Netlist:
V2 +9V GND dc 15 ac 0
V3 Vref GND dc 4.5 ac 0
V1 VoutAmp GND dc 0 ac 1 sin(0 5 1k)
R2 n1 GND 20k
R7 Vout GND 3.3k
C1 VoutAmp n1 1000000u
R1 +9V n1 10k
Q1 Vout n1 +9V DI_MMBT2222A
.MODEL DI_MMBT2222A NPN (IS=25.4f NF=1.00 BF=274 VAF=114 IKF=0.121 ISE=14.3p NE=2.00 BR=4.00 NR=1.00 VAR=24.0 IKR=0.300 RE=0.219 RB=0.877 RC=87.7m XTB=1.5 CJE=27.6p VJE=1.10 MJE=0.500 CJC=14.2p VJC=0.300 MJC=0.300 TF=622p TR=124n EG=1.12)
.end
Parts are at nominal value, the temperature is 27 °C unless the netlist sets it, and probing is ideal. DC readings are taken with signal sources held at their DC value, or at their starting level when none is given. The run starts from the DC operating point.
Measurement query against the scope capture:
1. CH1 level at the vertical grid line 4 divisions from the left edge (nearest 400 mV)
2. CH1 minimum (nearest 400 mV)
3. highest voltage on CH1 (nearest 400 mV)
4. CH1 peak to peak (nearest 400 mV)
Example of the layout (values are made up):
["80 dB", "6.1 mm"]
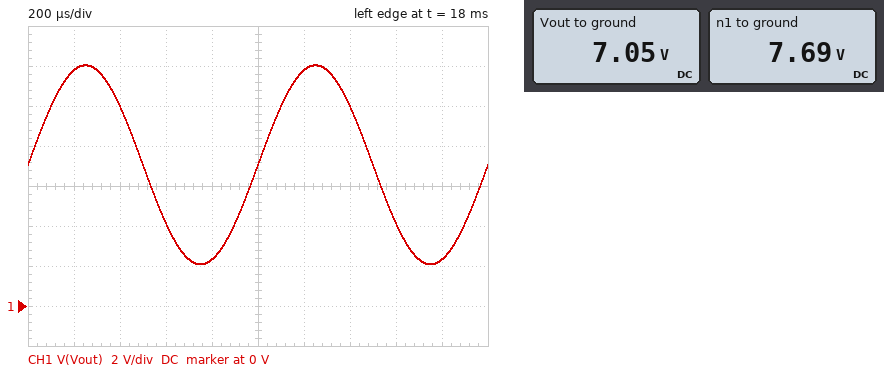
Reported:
["2.4 V", "2.0 V", "12.0 V", "10.0 V"]
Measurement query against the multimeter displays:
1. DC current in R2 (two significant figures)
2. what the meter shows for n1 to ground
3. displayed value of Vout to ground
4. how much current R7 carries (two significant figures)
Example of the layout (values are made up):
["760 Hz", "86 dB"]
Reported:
["380 µA", "7.69 V", "7.05 V", "2.1 mA"]
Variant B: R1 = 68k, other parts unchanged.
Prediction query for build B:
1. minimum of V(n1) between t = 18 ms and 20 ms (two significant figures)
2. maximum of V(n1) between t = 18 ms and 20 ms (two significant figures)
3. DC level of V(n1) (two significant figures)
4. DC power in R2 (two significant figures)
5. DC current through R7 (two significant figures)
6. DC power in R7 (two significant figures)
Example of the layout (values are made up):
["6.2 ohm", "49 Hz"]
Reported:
["-2.7 V", "7.3 V", "2.3 V", "260 µW", "510 µA", "870 µW"]
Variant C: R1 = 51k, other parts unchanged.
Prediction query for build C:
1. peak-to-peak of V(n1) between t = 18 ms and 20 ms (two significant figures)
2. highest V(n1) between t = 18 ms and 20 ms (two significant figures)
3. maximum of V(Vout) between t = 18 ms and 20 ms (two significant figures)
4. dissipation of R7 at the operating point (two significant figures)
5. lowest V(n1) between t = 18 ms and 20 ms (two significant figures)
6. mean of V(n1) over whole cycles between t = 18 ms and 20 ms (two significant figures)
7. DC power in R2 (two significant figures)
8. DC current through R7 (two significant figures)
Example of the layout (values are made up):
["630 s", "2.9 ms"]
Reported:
["10 V", "7.8 V", "7.2 V", "1.5 mW", "-2.2 V", "2.8 V", "400 µW", "680 µA"]
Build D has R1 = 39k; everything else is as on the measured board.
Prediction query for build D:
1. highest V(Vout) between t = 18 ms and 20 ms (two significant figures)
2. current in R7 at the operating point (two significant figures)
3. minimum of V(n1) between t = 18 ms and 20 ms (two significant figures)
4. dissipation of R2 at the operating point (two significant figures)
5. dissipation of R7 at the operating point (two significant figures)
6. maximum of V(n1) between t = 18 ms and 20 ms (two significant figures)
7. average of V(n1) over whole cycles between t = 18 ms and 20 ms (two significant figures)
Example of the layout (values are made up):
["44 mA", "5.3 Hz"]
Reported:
["7.8 V", "860 µA", "-1.6 V", "590 µW", "2.4 mW", "8.4 V", "3.4 V"]
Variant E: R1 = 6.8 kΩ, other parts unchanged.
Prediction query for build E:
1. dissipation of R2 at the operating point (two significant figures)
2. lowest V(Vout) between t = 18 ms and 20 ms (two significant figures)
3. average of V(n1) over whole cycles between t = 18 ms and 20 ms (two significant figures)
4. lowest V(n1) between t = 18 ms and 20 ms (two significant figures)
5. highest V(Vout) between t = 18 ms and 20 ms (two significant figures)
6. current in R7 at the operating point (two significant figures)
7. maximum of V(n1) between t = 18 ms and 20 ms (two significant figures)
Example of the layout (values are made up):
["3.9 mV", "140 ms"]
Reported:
["4.1 mW", "3.4 V", "9.0 V", "4.0 V", "13 V", "2.5 mA", "14 V"]
